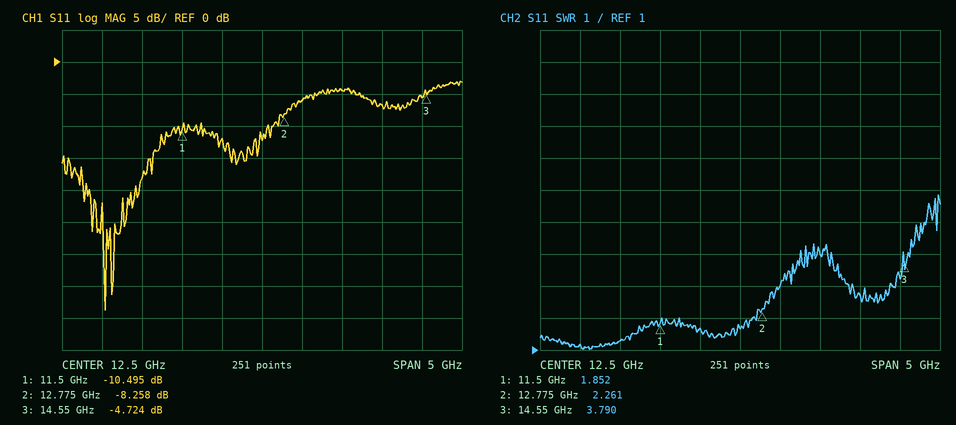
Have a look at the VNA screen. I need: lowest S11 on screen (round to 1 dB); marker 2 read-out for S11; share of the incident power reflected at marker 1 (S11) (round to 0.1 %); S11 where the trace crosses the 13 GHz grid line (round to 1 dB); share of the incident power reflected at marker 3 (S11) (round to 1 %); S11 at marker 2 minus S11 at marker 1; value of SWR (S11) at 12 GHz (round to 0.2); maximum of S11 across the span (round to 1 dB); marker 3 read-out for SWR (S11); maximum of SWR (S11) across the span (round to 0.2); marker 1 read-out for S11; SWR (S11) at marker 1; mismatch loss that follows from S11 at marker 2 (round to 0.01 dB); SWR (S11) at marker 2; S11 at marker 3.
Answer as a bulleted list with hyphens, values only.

- -39 dB
- -8.258 dB
- 8.9 %
- -6 dB
- 34 %
- 2.237 dB
- 1.6
- -3 dB
- 3.790
- 5.8
- -10.495 dB
- 1.852
- 0.70 dB
- 2.261
- -4.724 dB
